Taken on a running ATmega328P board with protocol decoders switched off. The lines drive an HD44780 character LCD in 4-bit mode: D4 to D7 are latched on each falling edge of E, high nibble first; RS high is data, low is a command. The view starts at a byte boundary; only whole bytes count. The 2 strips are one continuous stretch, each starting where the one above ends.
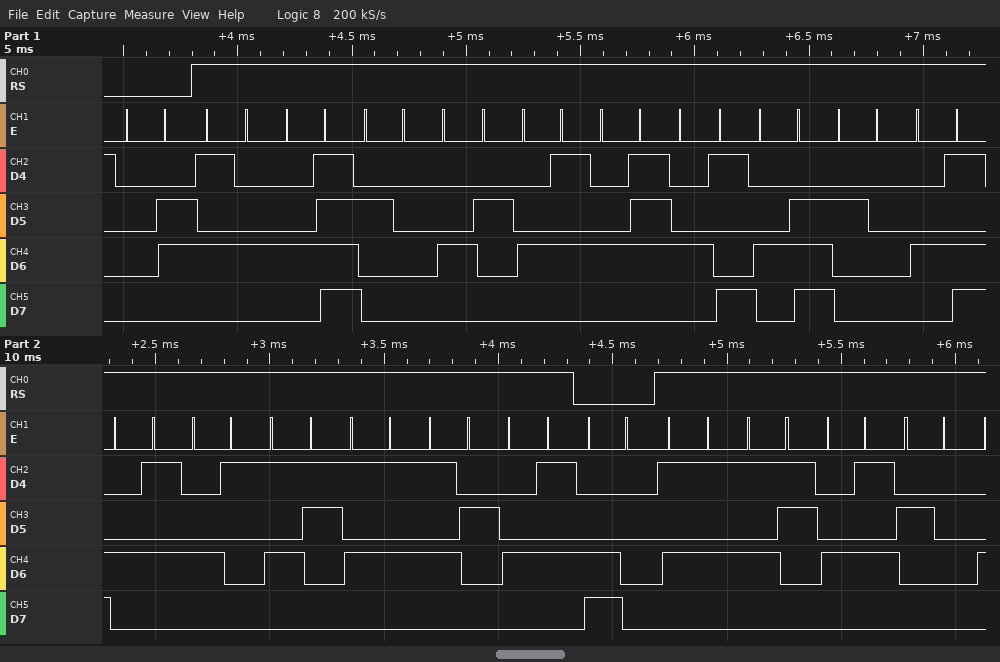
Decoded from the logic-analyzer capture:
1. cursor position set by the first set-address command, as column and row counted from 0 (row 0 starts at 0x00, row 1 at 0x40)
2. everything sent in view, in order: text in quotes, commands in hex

column 0, row 1
0x06 "TO BEGIN MEASURE" 0xC0 "USE "
